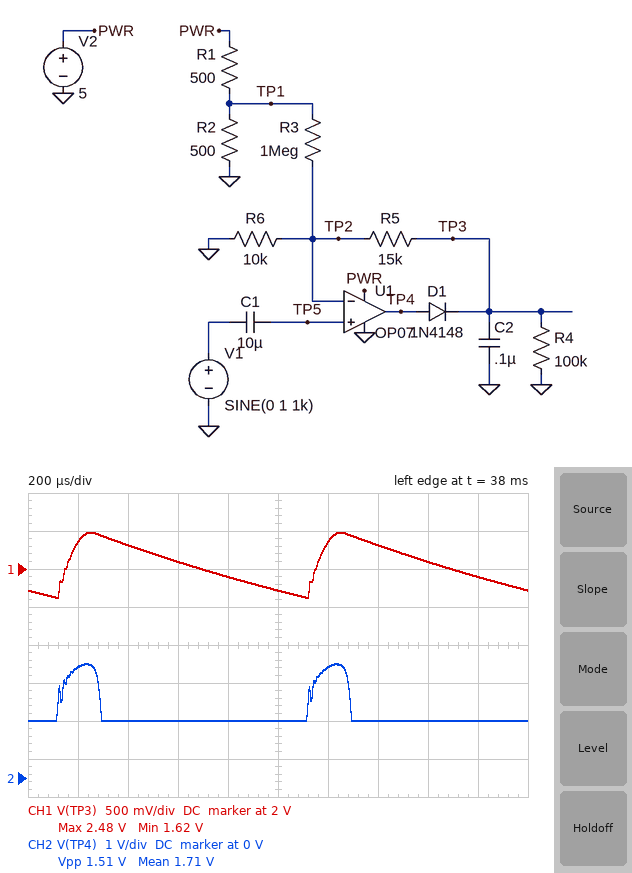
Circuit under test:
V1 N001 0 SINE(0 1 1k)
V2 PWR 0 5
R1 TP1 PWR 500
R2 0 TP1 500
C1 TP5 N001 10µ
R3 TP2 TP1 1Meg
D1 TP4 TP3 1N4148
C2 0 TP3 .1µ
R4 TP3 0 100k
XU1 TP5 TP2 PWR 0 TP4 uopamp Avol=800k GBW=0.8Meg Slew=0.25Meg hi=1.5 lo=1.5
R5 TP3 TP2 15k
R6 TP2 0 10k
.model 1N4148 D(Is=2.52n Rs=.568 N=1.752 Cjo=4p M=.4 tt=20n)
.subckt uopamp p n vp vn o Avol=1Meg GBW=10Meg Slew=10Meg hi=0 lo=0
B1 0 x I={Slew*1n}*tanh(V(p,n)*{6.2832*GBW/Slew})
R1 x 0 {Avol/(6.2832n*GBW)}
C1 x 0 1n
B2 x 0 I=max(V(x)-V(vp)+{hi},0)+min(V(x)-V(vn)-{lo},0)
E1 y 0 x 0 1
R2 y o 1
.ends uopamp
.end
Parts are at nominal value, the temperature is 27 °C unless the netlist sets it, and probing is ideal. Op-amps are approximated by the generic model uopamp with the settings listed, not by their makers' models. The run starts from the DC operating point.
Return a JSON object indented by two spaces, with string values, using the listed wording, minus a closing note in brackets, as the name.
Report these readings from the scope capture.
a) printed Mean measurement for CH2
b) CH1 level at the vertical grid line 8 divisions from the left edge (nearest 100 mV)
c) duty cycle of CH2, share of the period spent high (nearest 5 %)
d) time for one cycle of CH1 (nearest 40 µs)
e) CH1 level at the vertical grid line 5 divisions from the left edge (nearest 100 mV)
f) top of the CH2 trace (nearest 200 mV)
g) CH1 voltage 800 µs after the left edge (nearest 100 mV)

{
  "printed Mean measurement for CH2": "1.71 V",
  "CH1 level at the vertical grid line 8 divisions from the left edge": "2.1 V",
  "duty cycle of CH2, share of the period spent high": "15 %",
  "time for one cycle of CH1": "1.00 ms",
  "CH1 level at the vertical grid line 5 divisions from the left edge": "1.7 V",
  "top of the CH2 trace": "3.0 V",
  "CH1 voltage 800 µs after the left edge": "1.9 V"
}
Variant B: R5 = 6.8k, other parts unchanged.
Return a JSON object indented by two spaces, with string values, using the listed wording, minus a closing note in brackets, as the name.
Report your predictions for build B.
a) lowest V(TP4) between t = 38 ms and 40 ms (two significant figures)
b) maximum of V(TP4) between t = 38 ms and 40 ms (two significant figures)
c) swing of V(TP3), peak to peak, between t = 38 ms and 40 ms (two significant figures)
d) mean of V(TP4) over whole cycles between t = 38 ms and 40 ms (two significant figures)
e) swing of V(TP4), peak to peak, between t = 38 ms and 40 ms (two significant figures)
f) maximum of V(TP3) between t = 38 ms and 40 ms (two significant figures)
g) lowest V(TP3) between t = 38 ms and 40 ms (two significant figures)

{
  "lowest V(TP4) between t = 38 ms and 40 ms": "1.5 V",
  "maximum of V(TP4) between t = 38 ms and 40 ms": "2.2 V",
  "swing of V(TP3), peak to peak, between t = 38 ms and 40 ms": "630 mV",
  "mean of V(TP4) over whole cycles between t = 38 ms and 40 ms": "1.6 V",
  "swing of V(TP4), peak to peak, between t = 38 ms and 40 ms": "680 mV",
  "maximum of V(TP3) between t = 38 ms and 40 ms": "1.7 V",
  "lowest V(TP3) between t = 38 ms and 40 ms": "1.0 V"
}
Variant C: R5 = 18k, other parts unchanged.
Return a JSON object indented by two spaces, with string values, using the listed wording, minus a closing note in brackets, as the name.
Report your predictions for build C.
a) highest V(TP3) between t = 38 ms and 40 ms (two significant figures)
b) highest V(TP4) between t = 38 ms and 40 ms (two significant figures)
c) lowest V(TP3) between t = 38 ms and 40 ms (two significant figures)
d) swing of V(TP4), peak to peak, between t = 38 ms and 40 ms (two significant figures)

{
  "highest V(TP3) between t = 38 ms and 40 ms": "2.8 V",
  "highest V(TP4) between t = 38 ms and 40 ms": "3.3 V",
  "lowest V(TP3) between t = 38 ms and 40 ms": "1.9 V",
  "swing of V(TP4), peak to peak, between t = 38 ms and 40 ms": "1.8 V"
}
